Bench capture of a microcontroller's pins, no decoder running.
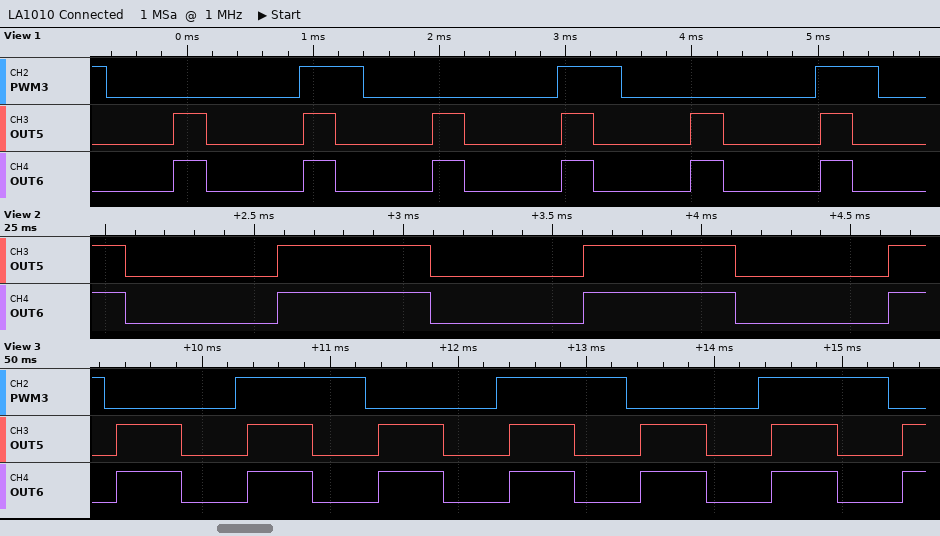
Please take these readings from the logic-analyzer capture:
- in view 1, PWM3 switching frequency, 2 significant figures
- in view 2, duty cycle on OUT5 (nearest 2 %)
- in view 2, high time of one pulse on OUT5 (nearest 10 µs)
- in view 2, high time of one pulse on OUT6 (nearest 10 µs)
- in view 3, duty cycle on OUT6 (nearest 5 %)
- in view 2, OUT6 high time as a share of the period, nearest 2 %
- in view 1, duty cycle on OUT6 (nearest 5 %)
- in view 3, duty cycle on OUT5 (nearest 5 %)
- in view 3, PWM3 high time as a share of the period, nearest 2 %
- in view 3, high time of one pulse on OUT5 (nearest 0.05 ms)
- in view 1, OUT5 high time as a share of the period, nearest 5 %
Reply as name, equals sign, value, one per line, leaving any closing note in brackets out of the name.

in view 1, PWM3 switching frequency, 2 significant figures = 490 Hz
in view 2, duty cycle on OUT5 = 50 %
in view 2, high time of one pulse on OUT5 = 510 µs
in view 2, high time of one pulse on OUT6 = 510 µs
in view 3, duty cycle on OUT6 = 50 %
in view 2, OUT6 high time as a share of the period, nearest 2 % = 50 %
in view 1, duty cycle on OUT6 = 25 %
in view 3, duty cycle on OUT5 = 50 %
in view 3, PWM3 high time as a share of the period, nearest 2 % = 50 %
in view 3, high time of one pulse on OUT5 = 0.50 ms
in view 1, OUT5 high time as a share of the period, nearest 5 % = 25 %
